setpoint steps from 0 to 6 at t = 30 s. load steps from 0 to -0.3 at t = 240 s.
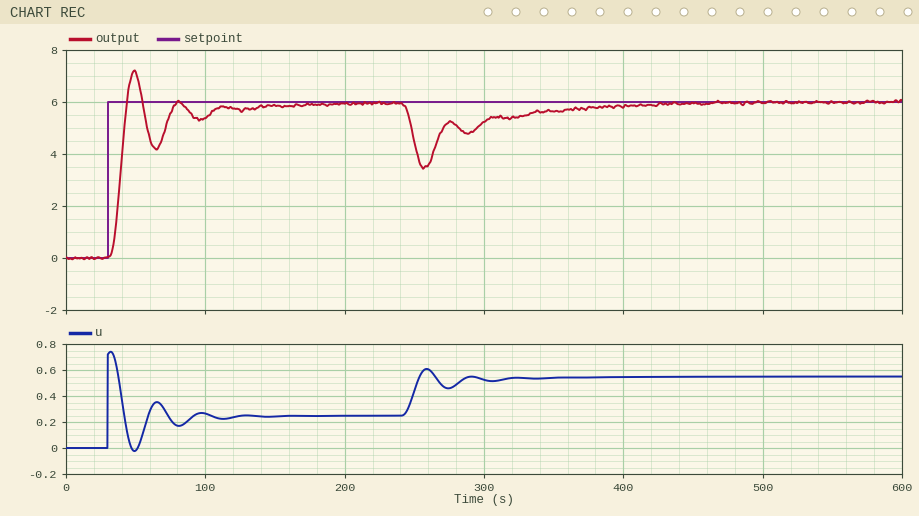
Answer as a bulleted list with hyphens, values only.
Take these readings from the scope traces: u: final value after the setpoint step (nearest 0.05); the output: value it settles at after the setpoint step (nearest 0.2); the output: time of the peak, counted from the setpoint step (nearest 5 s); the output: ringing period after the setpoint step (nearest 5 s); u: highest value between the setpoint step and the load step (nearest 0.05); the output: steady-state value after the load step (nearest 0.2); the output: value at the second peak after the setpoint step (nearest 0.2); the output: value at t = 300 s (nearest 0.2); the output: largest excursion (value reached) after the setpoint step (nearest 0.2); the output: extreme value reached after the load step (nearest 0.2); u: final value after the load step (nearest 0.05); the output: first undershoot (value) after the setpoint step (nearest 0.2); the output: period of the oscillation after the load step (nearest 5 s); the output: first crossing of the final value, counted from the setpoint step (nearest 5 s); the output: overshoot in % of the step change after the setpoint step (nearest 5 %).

- 0.25
- 6.0
- 20 s
- 30 s
- 0.75
- 6.0
- 6.0
- 5.2
- 7.2
- 3.4
- 0.55
- 4.2
- 30 s
- 15 s
- 20 %
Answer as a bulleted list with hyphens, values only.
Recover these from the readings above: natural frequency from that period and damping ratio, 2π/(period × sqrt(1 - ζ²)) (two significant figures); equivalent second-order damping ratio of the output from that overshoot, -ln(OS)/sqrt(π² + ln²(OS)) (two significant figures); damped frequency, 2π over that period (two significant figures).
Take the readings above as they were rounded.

- 0.24 rad/s
- 0.46
- 0.21 rad/s
